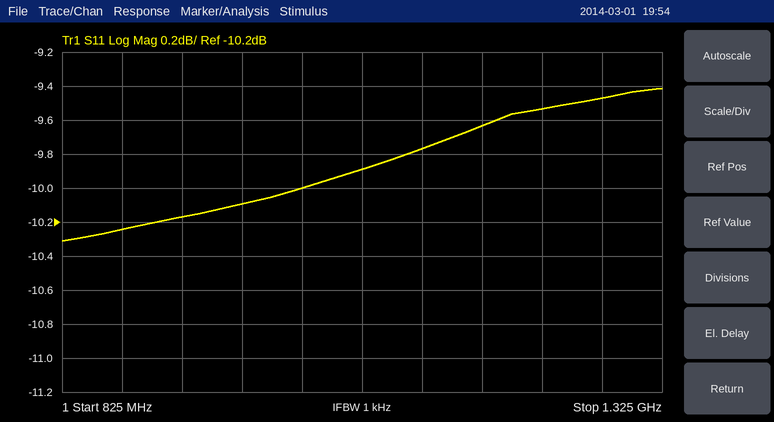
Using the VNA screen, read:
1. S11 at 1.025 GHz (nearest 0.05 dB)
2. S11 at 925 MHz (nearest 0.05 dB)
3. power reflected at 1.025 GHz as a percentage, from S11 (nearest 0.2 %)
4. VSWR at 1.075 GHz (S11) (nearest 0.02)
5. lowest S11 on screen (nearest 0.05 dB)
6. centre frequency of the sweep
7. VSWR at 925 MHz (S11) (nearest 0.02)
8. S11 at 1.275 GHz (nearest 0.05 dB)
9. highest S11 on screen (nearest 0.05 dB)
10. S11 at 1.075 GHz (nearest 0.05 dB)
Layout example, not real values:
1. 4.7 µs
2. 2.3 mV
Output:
1. -10.00 dB
2. -10.15 dB
3. 10.0 %
4. 1.94
5. -10.30 dB
6. 1.075 GHz
7. 1.90
8. -9.45 dB
9. -9.40 dB
10. -9.90 dB
